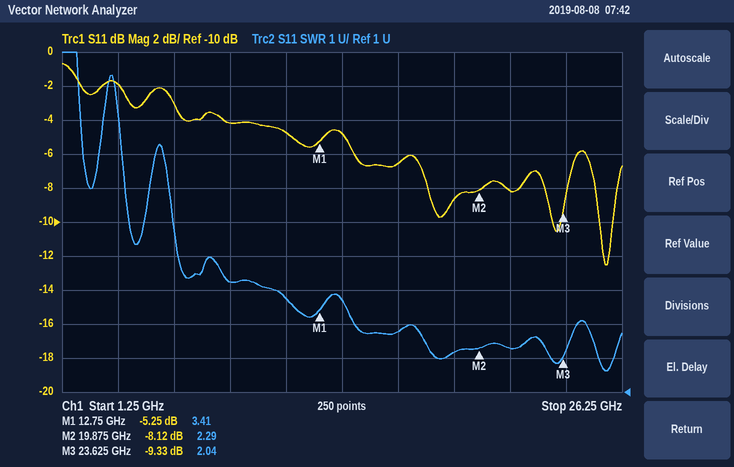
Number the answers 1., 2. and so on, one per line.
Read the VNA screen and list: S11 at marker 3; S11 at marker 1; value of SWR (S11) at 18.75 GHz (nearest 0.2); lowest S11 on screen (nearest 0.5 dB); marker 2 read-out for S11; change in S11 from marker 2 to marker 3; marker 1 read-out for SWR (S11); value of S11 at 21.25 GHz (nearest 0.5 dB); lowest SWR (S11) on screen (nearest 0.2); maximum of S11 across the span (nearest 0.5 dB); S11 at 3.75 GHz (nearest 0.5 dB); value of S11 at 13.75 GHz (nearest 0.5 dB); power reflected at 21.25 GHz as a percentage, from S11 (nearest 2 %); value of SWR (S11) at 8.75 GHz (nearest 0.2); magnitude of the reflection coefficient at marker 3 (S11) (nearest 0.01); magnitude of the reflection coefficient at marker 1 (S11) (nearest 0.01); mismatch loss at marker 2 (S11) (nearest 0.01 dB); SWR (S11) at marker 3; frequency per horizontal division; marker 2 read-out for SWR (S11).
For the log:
1. -9.33 dB
2. -5.25 dB
3. 2.2
4. -12.5 dB
5. -8.12 dB
6. -1.21 dB
7. 3.41
8. -8.0 dB
9. 1.6
10. -0.5 dB
11. -2.0 dB
12. -5.0 dB
13. 16 %
14. 4.2
15. 0.34
16. 0.55
17. 0.73 dB
18. 2.04
19. 2.5 GHz
20. 2.29
